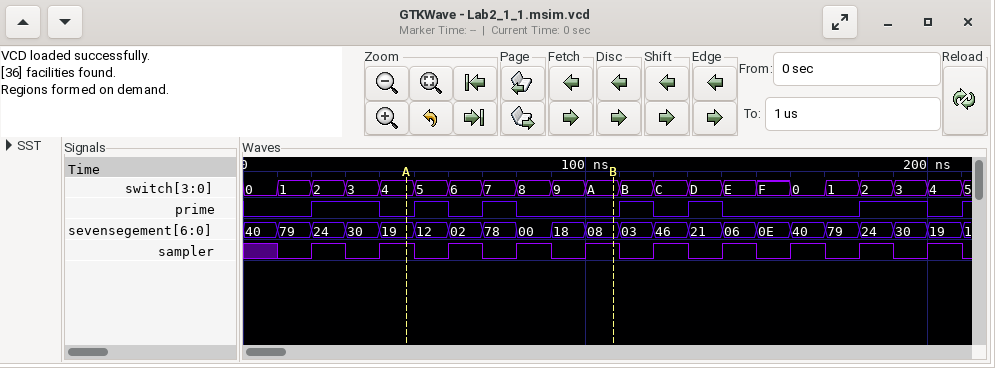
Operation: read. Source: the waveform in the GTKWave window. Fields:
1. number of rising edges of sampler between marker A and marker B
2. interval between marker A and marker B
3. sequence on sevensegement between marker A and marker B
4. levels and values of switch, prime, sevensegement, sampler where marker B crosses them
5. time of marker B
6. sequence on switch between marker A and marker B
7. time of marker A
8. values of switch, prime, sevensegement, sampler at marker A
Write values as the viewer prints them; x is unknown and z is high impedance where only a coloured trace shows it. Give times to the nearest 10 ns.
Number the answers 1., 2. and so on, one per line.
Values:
1. 3
2. 60 ns
3. 19, 12, 02, 78, 00, 18, 08
4. switch=A, prime=0, sevensegement=08, sampler=1
5. 110 ns
6. 4, 5, 6, 7, 8, 9, A
7. 50 ns
8. switch=4, prime=0, sevensegement=19, sampler=1
